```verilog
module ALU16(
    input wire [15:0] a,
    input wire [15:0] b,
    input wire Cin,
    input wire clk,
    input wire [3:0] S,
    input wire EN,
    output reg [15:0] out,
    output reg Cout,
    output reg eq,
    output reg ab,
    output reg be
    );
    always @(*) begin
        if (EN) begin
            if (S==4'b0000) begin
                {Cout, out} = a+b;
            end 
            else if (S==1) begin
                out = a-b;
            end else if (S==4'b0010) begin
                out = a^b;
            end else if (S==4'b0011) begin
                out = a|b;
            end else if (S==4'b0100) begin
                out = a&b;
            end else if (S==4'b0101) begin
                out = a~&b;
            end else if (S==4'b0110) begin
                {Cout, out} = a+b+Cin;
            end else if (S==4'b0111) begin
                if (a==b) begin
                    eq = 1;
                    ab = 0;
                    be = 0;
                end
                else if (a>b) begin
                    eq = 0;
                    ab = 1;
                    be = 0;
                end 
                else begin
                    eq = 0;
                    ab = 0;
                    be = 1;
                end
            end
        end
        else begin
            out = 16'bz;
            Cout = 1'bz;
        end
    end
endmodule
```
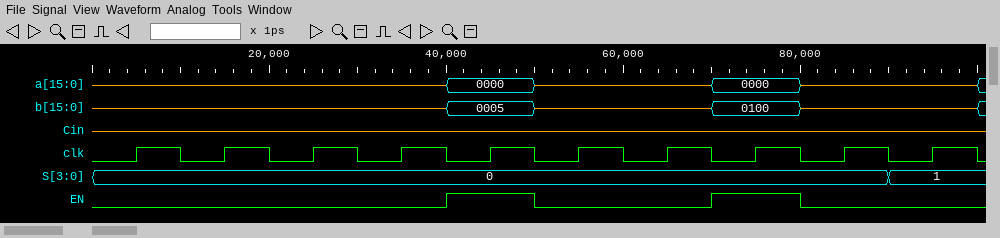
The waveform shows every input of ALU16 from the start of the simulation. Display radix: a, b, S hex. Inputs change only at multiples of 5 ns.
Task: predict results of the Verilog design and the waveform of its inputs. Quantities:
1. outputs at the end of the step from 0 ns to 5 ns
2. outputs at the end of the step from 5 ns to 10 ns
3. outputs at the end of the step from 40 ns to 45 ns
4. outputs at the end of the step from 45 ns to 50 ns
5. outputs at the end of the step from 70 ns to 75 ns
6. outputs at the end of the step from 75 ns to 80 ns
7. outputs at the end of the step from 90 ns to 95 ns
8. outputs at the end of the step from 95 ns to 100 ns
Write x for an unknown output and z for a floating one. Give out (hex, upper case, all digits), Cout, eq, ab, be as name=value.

out=z, Cout=z, eq=x, ab=x, be=x
out=z, Cout=z, eq=x, ab=x, be=x
out=0005, Cout=0, eq=x, ab=x, be=x
out=0005, Cout=0, eq=x, ab=x, be=x
out=0100, Cout=0, eq=x, ab=x, be=x
out=0100, Cout=0, eq=x, ab=x, be=x
out=z, Cout=z, eq=x, ab=x, be=x
out=z, Cout=z, eq=x, ab=x, be=x
